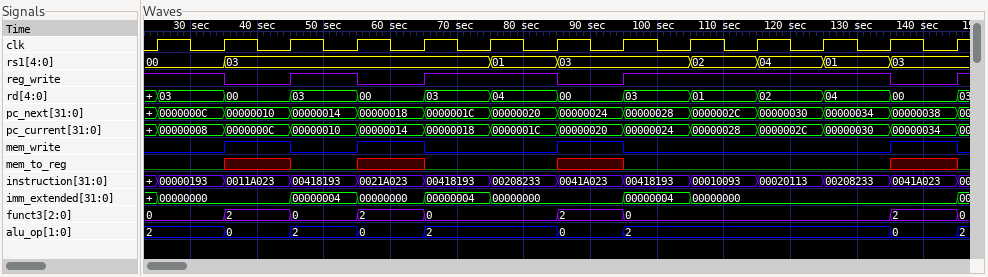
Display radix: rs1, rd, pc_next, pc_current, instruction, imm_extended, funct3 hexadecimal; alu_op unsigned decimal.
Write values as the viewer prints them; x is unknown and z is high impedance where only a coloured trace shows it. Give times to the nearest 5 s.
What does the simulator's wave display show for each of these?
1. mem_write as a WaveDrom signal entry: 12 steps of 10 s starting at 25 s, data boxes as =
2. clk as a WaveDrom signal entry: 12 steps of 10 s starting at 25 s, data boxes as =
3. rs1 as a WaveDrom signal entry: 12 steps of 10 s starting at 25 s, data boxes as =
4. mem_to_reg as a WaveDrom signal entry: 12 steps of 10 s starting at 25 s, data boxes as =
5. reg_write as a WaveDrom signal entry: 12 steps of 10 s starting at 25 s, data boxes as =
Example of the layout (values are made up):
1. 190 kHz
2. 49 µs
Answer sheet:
1. {name: 'mem_write', wave: '01010.10...1'}
2. {name: 'clk', wave: 'p...........'}
3. {name: 'rs1', wave: '==...==.====', data: '00 03 01 03 02 04 01 03'}
4. {name: 'mem_to_reg', wave: '0x0x0.x0...x'}
5. {name: 'reg_write', wave: '10101.01...0'}
